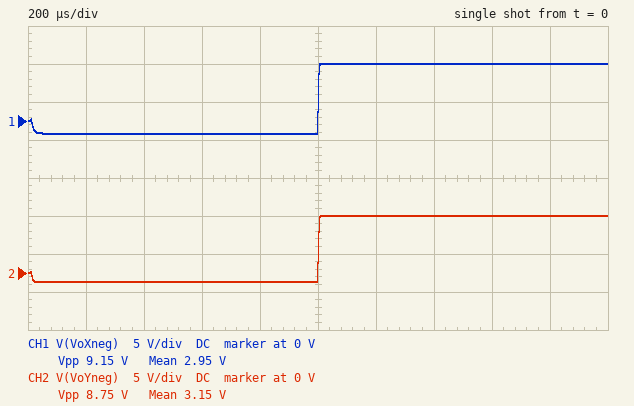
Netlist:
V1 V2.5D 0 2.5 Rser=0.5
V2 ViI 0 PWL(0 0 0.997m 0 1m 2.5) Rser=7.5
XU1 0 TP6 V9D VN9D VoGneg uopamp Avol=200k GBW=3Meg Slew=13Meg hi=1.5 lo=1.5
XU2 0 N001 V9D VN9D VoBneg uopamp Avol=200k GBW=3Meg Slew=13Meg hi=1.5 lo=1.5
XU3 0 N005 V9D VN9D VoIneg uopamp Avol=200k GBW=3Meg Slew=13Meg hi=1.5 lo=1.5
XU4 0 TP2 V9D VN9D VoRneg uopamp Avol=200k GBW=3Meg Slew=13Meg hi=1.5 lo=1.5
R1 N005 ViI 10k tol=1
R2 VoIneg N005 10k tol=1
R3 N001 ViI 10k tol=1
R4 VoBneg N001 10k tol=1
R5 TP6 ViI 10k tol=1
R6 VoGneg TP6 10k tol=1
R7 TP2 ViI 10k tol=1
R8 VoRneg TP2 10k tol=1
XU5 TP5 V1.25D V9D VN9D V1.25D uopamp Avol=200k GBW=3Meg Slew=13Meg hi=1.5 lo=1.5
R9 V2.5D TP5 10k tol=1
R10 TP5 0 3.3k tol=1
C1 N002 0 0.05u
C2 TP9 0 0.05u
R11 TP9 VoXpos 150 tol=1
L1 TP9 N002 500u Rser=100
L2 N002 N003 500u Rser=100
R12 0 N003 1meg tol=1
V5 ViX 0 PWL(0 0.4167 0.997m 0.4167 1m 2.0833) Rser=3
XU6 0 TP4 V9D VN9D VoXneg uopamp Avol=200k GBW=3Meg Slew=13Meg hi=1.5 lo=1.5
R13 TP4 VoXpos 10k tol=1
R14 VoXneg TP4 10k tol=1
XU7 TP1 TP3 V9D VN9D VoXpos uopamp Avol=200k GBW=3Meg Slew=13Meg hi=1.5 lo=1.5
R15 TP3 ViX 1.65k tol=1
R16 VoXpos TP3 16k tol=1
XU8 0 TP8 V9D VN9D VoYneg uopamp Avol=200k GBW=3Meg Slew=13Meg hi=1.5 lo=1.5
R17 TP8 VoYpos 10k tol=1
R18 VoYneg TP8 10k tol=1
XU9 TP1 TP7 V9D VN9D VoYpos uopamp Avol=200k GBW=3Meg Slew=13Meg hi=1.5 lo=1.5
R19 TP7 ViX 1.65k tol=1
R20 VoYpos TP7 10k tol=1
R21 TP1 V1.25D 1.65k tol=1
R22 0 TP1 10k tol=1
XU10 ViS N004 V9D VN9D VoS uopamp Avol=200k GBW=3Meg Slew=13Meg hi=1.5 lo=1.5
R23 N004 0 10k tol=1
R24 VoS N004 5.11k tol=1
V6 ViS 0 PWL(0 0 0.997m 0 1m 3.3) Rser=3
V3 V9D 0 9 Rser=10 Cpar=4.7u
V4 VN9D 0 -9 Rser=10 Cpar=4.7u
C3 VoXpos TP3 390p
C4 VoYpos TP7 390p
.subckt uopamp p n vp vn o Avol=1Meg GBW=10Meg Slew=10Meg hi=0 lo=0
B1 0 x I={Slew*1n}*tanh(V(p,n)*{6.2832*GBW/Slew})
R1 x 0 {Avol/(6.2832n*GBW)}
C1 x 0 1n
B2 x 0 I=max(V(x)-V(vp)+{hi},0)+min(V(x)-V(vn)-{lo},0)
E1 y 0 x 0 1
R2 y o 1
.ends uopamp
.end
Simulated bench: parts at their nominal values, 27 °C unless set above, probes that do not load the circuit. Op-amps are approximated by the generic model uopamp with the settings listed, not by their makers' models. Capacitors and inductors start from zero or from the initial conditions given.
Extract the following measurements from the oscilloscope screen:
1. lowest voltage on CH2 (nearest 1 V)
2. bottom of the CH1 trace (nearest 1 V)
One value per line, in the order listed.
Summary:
-1 V
-2 V
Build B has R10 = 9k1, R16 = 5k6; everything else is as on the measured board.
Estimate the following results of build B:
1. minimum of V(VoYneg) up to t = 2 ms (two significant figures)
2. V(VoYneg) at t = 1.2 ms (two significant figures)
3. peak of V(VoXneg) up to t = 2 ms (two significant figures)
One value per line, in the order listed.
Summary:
-4.7 V
5.4 V
2.6 V
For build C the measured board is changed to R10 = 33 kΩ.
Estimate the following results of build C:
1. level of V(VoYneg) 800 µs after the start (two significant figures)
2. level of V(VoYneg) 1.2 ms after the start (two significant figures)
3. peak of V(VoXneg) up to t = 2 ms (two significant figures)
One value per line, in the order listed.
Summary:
-7.5 V
990 mV
2.6 V
